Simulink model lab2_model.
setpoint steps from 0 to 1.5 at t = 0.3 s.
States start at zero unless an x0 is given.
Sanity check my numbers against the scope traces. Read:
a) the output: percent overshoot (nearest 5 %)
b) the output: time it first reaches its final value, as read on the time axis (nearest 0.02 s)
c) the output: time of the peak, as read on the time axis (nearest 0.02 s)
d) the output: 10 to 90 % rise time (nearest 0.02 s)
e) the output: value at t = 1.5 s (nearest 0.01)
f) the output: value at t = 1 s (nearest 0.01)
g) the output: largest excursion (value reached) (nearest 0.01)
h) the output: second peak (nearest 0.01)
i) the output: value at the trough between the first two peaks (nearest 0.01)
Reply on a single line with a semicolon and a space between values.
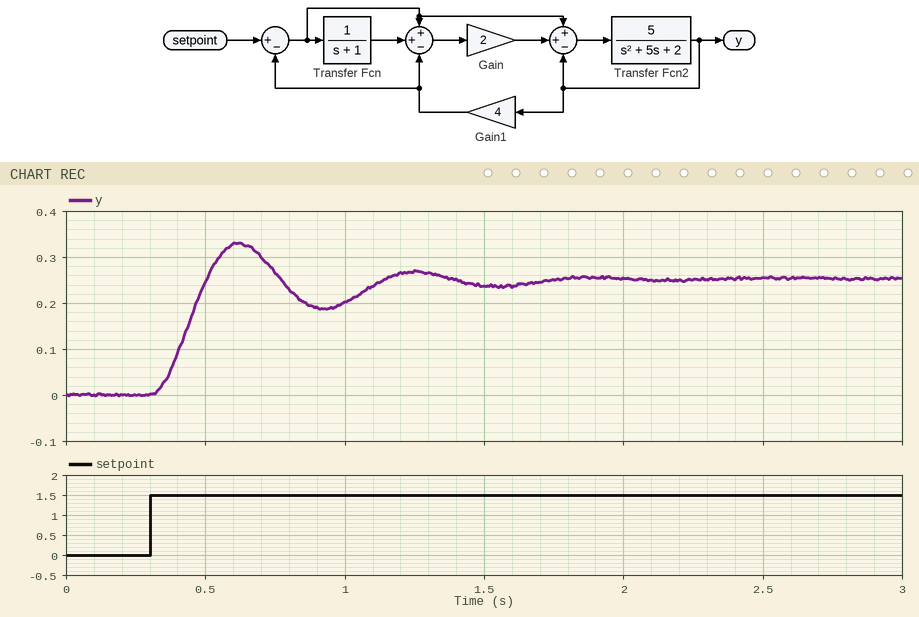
30 %; 0.50 s; 0.62 s; 0.14 s; 0.24; 0.20; 0.33; 0.27; 0.19
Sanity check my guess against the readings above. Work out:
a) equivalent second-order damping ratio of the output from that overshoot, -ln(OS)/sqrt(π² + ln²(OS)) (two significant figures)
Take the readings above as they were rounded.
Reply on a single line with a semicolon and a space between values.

0.36
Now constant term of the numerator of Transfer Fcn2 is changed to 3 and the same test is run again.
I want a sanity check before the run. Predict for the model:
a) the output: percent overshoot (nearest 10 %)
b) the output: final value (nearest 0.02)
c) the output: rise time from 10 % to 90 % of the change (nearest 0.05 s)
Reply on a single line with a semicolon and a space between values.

20 %; 0.26; 0.20 s
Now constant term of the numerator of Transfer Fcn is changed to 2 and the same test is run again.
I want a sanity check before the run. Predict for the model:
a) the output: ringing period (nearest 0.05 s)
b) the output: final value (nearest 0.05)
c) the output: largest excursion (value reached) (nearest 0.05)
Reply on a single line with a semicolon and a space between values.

0.65 s; 0.30; 0.35
